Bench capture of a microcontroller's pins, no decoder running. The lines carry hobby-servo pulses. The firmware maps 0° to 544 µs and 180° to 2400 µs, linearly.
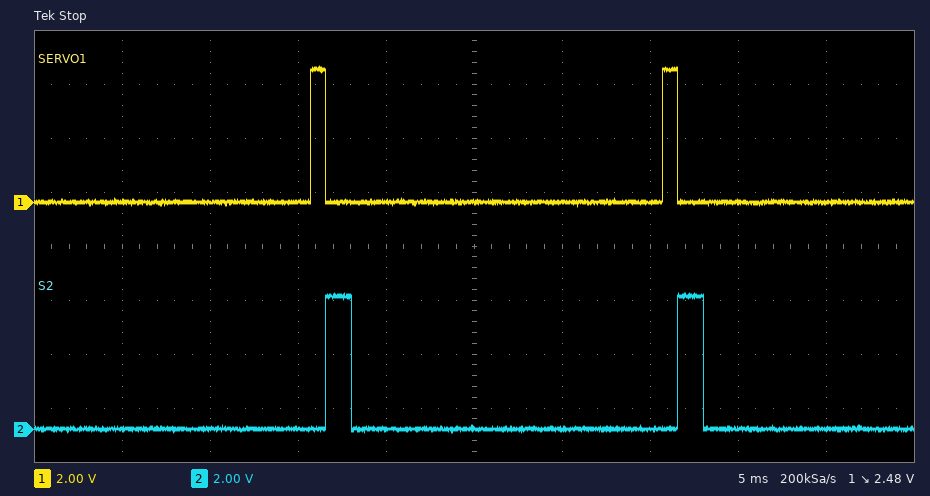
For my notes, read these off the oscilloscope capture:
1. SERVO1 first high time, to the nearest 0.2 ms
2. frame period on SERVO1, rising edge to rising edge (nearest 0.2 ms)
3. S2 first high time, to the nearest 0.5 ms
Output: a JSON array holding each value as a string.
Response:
["0.8 ms", "20.0 ms", "1.5 ms"]
